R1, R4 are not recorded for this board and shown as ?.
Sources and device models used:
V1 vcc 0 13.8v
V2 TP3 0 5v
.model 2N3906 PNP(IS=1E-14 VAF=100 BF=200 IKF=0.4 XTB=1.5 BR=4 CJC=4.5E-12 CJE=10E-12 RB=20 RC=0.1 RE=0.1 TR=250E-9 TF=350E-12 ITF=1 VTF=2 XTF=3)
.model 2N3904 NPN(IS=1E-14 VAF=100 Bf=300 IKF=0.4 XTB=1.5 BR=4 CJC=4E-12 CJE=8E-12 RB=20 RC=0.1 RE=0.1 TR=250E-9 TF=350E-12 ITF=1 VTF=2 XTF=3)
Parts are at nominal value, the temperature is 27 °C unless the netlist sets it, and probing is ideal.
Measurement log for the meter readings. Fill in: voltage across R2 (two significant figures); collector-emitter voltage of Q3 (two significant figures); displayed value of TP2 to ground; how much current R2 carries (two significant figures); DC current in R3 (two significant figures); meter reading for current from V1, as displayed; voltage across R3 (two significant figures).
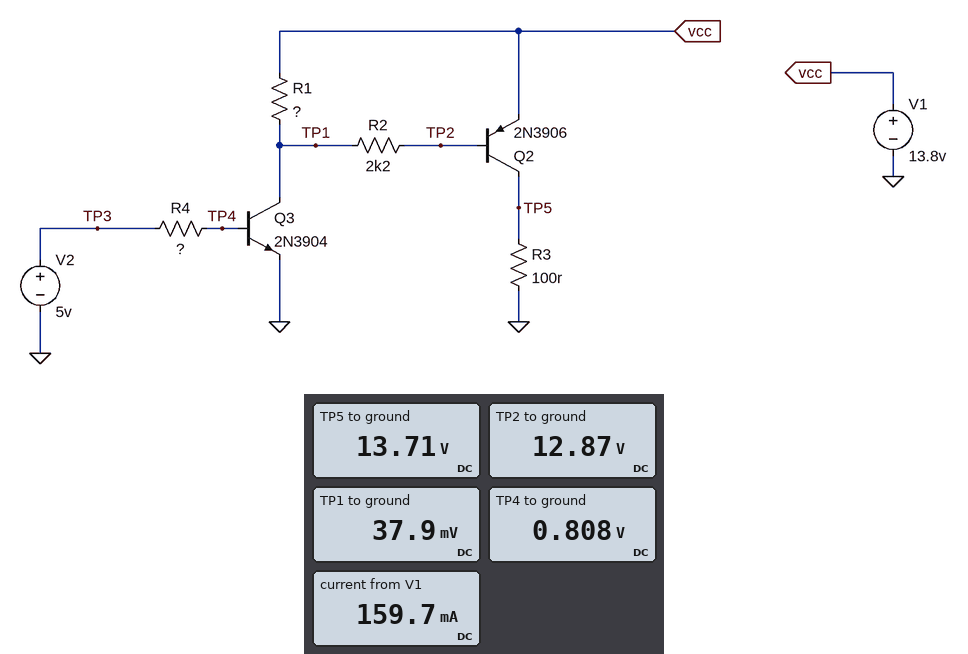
13 V
38 mV
12.87 V
5.8 mA
140 mA
159.7 mA
14 V
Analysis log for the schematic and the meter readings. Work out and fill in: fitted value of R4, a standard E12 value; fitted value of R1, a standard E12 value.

1.5 kΩ
820 Ω
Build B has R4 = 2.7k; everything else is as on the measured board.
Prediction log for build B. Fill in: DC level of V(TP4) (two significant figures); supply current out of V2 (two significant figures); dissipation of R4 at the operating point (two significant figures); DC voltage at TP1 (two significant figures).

780 mV
1.6 mA
6.6 mW
49 mV
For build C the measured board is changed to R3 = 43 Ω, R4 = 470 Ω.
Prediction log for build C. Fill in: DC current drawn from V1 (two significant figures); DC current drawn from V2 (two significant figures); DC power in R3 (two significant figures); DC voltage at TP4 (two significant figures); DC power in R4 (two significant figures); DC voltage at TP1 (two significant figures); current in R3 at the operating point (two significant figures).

340 mA
8.6 mA
4.3 W
940 mV
35 mW
24 mV
320 mA
